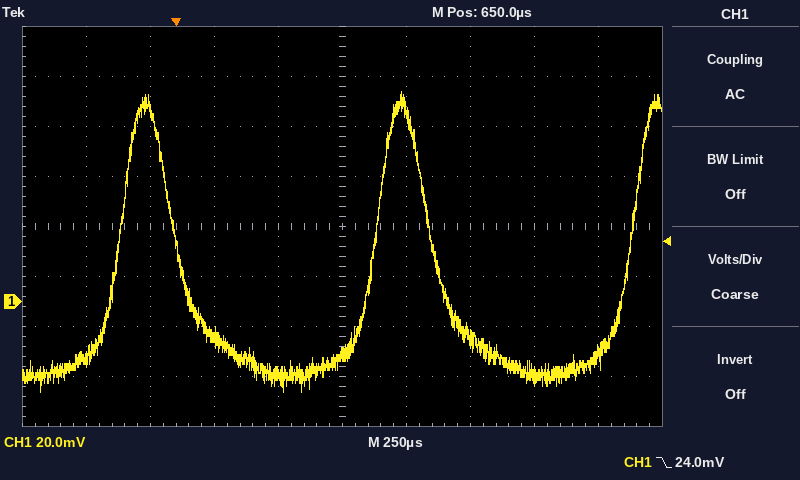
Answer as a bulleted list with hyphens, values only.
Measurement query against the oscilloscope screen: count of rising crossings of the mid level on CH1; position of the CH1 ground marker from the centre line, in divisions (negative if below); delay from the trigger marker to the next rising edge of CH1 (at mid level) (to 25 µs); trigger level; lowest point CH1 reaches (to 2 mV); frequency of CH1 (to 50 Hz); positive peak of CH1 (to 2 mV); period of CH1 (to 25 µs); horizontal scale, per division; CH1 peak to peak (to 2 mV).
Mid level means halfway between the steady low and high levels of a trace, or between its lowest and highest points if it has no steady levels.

- 3
- -1.5 div
- 775 µs
- 24.0 mV
- -36 mV
- 1.00 kHz
- 84 mV
- 1.000 ms
- 250 µs
- 120 mV
